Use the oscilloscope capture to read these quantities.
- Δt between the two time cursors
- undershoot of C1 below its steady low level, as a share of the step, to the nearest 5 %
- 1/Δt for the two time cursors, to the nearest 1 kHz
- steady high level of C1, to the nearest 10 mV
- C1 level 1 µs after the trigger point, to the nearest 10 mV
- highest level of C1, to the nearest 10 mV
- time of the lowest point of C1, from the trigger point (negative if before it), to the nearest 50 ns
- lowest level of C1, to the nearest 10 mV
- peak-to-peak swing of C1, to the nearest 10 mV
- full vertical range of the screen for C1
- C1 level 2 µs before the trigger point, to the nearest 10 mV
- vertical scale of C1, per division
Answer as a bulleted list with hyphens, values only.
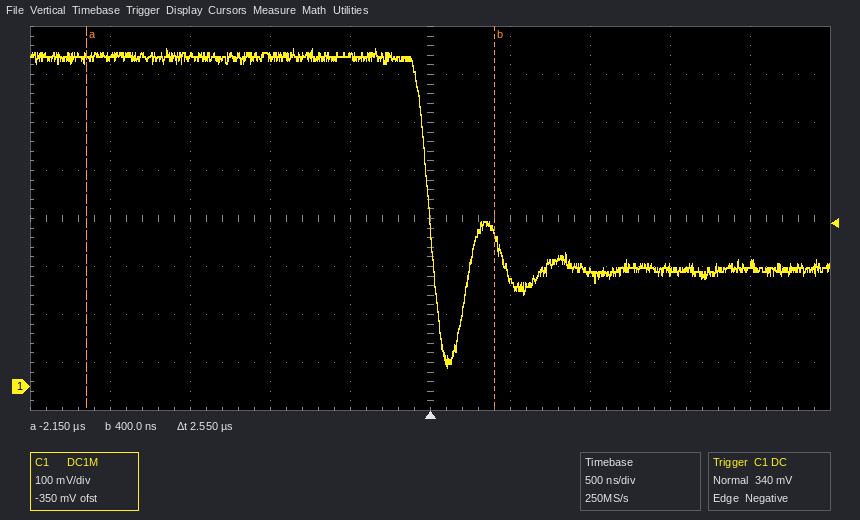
- 2.55 µs
- 45 %
- 392 kHz
- 690 mV
- 240 mV
- 700 mV
- +100 ns
- 40 mV
- 660 mV
- 800 mV
- 690 mV
- 100 mV
